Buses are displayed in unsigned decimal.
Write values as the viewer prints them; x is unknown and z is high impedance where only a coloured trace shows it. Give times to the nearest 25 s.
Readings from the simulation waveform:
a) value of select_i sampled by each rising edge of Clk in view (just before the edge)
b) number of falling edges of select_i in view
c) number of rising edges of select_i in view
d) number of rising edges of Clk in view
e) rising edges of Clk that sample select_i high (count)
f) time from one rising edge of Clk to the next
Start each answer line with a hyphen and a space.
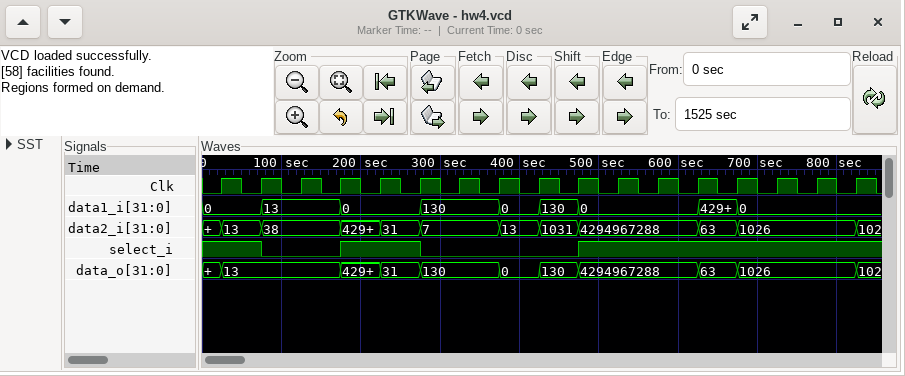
- 1 1 0 0 1 1 0 0 0 0 1 1 1 1 1 1 1
- 2
- 2
- 17
- 11
- 50 s
